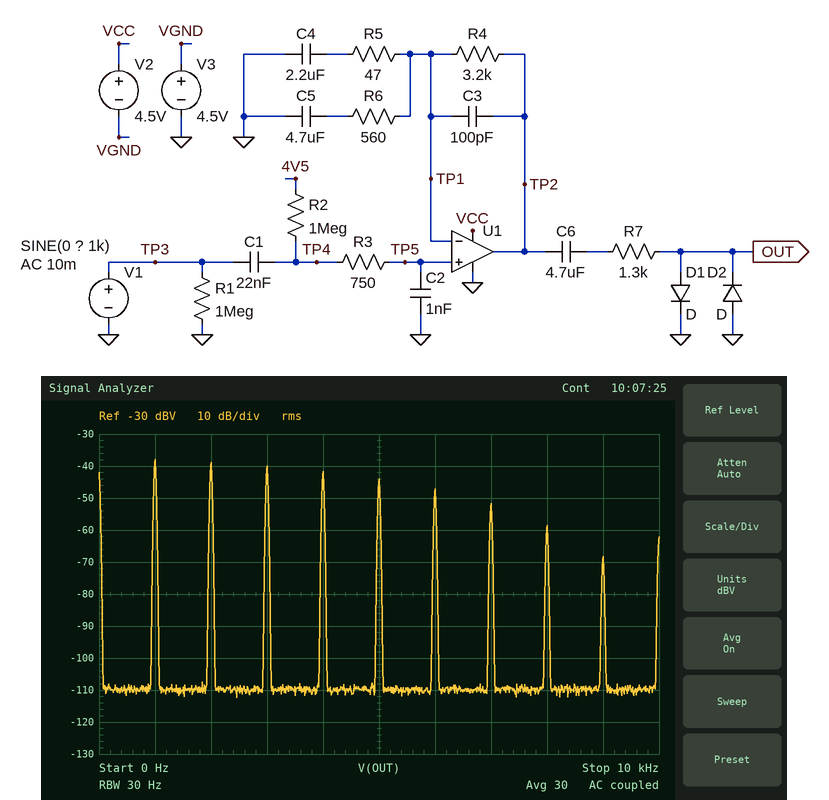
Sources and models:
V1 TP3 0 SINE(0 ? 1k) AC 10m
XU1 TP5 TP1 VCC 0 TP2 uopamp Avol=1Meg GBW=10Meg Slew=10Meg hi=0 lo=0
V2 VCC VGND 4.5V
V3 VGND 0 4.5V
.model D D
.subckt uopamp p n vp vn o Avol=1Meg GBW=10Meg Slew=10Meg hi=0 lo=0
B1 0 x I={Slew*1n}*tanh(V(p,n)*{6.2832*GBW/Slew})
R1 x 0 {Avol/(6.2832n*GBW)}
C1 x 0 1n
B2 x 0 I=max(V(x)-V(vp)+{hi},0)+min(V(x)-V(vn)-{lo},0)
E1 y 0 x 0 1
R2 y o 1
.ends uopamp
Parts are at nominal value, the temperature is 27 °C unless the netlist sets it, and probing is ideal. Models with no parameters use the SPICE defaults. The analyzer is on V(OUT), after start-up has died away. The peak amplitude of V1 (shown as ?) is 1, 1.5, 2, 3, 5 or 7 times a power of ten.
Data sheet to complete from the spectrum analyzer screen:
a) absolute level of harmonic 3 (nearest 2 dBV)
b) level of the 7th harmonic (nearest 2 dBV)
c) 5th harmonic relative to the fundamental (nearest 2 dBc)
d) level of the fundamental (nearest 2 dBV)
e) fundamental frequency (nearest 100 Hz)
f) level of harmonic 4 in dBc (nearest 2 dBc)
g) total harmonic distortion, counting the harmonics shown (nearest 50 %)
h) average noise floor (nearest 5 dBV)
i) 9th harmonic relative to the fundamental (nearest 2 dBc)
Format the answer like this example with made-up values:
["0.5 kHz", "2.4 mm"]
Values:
["-40 dBV", "-52 dBV", "-6 dBc", "-38 dBV", "1.0 kHz", "-4 dBc", "150 %", "-110 dBV", "-30 dBc"]
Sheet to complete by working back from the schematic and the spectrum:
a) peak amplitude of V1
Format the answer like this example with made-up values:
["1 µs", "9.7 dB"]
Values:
["10 mV"]
